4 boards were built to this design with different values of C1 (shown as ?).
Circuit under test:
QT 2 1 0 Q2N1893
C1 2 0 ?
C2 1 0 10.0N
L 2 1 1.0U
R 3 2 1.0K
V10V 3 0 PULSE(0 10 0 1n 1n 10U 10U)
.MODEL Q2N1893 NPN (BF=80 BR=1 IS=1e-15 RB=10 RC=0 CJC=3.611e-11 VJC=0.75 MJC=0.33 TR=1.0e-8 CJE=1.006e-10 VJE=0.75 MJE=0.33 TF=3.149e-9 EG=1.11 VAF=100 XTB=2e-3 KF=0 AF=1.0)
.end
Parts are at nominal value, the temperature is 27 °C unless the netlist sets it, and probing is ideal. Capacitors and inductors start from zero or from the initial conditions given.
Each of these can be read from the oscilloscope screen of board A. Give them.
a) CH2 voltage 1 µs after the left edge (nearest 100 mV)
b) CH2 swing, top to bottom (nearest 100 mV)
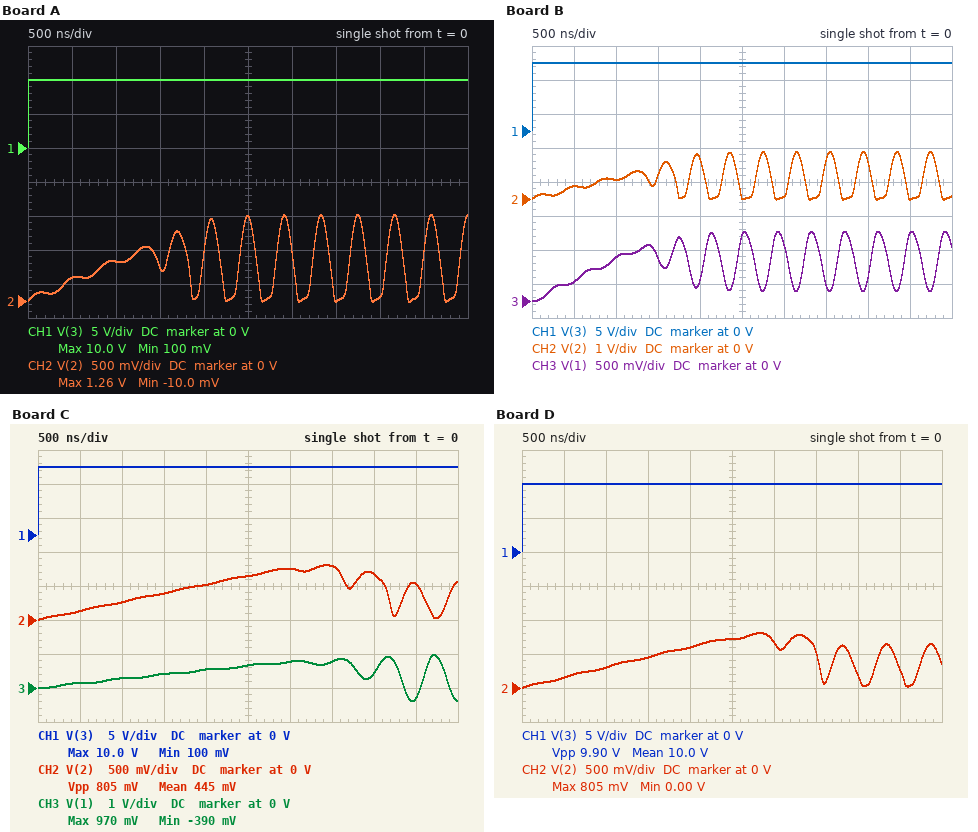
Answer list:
600 mV
1.3 V
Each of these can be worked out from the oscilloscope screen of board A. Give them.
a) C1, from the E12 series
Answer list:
6.8 nF
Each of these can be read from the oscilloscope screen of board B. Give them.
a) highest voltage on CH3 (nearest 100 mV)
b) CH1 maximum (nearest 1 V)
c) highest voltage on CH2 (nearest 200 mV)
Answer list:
1.0 V
10 V
1.4 V
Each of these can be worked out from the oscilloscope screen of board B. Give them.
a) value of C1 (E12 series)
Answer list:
5.6 nF
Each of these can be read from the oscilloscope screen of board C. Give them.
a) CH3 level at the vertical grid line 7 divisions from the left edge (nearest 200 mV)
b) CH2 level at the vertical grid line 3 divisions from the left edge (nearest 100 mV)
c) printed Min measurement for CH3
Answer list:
800 mV
400 mV
-390 mV
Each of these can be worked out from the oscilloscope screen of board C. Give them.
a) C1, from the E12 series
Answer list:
27 nF
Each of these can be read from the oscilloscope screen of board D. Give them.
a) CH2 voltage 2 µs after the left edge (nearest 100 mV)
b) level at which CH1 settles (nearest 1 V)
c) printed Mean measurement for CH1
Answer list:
600 mV
10 V
10.0 V
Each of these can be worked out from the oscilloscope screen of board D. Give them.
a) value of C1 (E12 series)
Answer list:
22 nF
